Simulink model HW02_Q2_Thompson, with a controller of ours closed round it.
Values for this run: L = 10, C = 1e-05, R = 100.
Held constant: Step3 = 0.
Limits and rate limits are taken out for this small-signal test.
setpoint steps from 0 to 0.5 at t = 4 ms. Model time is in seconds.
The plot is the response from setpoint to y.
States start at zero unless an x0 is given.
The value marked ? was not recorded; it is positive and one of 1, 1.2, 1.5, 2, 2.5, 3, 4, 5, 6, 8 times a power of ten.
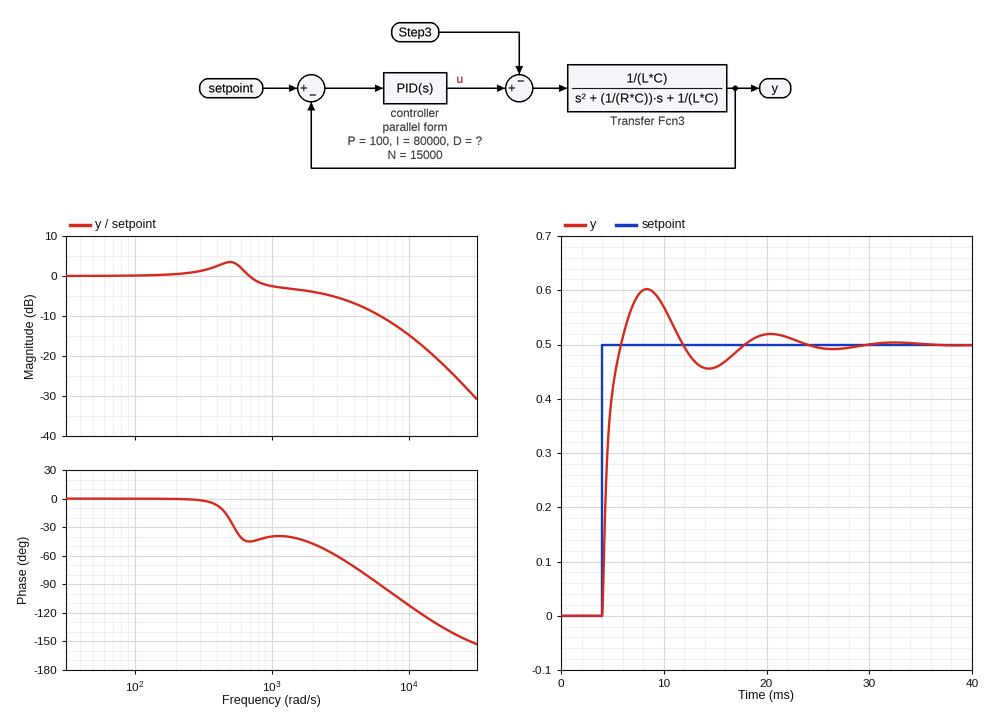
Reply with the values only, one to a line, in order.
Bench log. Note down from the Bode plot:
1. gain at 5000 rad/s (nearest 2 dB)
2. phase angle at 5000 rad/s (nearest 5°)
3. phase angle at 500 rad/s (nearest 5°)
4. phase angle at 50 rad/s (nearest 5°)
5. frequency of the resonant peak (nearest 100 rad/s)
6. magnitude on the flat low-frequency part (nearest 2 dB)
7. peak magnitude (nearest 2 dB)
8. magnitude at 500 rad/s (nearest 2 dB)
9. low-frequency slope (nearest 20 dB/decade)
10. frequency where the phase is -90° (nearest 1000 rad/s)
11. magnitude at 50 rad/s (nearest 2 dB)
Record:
-8 dB
-80°
-25°
0°
500 rad/s
0 dB
4 dB
4 dB
0 dB/decade
6000 rad/s
0 dB
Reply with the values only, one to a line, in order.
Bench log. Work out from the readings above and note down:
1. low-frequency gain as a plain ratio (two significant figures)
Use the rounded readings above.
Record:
1.0
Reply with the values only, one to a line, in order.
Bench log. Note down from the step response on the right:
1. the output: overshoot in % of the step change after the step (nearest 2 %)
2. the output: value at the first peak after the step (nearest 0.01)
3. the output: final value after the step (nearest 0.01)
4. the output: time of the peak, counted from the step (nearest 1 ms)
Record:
20 %
0.60
0.50
4 ms
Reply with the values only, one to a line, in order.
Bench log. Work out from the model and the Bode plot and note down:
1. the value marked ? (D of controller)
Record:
0.2
